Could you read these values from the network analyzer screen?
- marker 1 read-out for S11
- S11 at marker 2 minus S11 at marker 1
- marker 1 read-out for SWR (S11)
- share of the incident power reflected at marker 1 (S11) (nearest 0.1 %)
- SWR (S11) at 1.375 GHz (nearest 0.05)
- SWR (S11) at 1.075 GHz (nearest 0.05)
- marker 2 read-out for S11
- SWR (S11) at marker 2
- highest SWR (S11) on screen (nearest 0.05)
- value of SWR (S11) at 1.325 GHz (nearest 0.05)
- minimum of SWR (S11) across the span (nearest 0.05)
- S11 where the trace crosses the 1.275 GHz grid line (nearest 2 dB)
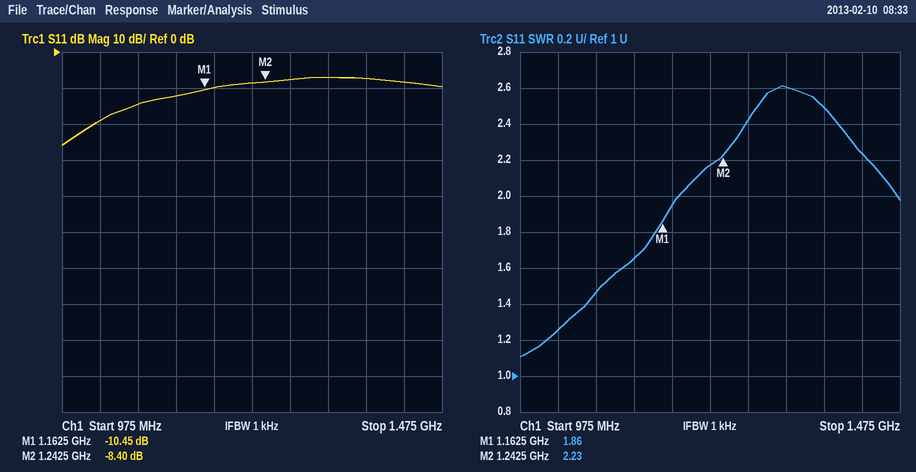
-10.45 dB
2.05 dB
1.86
9.0 %
2.50
1.45
-8.40 dB
2.23
2.60
2.60
1.10
-8 dB
